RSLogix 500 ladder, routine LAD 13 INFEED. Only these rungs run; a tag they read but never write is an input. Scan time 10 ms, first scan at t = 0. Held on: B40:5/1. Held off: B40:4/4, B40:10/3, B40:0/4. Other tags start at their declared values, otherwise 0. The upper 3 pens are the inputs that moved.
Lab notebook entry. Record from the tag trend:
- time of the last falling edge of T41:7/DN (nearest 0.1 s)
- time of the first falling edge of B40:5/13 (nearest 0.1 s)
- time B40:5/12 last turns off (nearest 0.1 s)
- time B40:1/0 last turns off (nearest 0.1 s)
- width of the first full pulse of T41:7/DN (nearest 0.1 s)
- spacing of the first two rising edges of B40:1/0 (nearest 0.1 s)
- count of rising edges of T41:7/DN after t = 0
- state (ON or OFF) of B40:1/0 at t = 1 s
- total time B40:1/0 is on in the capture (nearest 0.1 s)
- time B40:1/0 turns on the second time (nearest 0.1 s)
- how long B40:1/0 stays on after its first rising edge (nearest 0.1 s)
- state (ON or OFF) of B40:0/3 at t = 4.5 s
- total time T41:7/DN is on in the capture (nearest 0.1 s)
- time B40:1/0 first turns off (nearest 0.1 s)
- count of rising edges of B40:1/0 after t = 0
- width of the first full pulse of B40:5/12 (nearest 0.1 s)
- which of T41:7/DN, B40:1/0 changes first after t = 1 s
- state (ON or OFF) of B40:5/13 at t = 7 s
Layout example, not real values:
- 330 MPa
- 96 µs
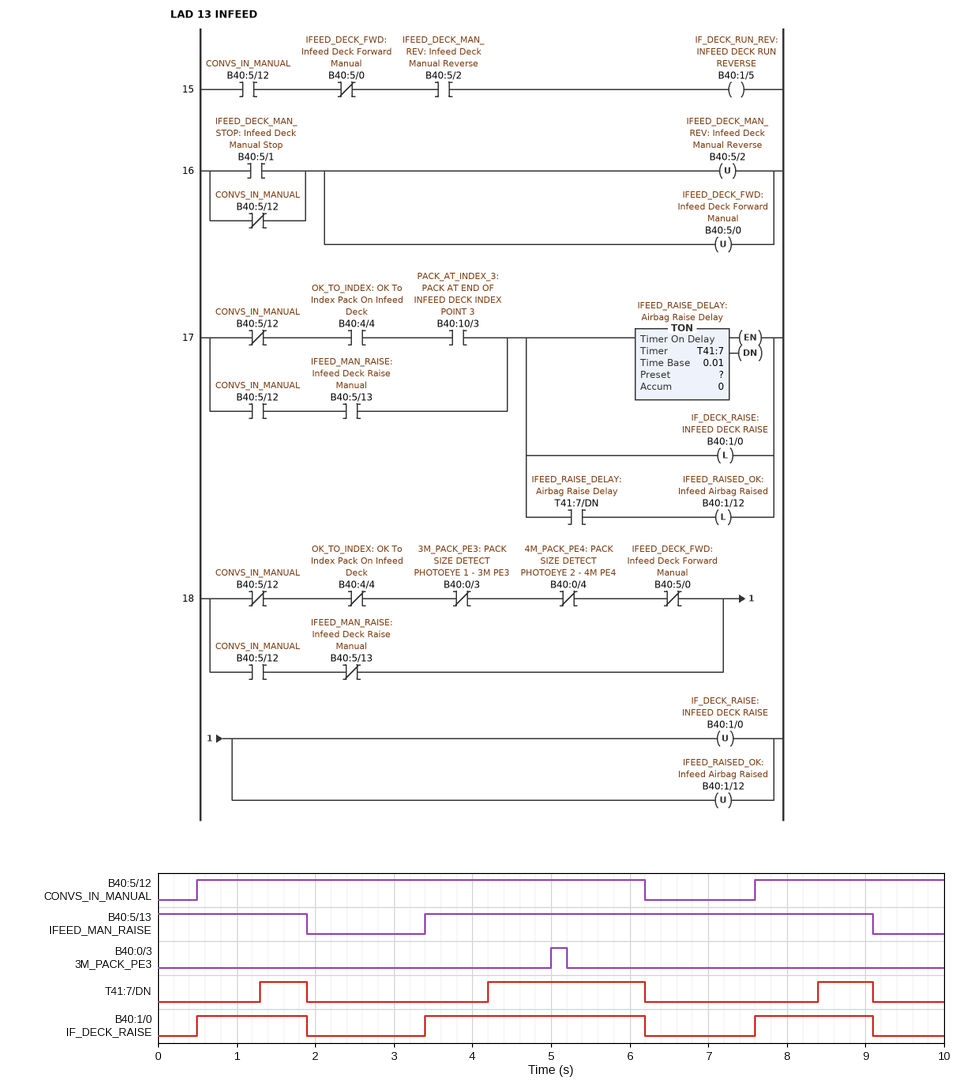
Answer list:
- 9.1 s
- 1.9 s
- 6.2 s
- 9.1 s
- 0.6 s
- 2.9 s
- 3
- ON
- 5.7 s
- 3.4 s
- 1.4 s
- OFF
- 3.3 s
- 1.9 s
- 3
- 5.7 s
- T41:7/DN
- ON
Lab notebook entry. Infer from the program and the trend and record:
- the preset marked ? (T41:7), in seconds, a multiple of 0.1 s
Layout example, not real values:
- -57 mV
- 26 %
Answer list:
- 0.8 s
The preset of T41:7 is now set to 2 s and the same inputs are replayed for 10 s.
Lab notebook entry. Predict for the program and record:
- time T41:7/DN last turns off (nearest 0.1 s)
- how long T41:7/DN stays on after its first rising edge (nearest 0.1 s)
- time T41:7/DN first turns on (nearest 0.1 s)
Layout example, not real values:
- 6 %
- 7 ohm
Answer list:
- 6.2 s
- 0.8 s
- 5.4 s
